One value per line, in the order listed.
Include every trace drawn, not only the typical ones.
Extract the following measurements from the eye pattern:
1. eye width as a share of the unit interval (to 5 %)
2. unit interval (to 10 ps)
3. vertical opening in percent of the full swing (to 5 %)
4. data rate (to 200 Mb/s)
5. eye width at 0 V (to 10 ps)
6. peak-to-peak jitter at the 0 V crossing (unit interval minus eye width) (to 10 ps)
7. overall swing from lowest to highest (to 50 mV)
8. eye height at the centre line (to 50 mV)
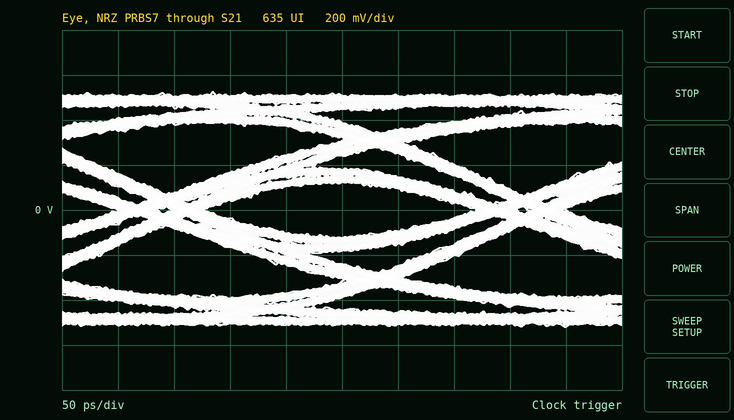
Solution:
75 %
320 ps
25 %
3.2 Gb/s
240 ps
80 ps
1.05 V
250 mV
